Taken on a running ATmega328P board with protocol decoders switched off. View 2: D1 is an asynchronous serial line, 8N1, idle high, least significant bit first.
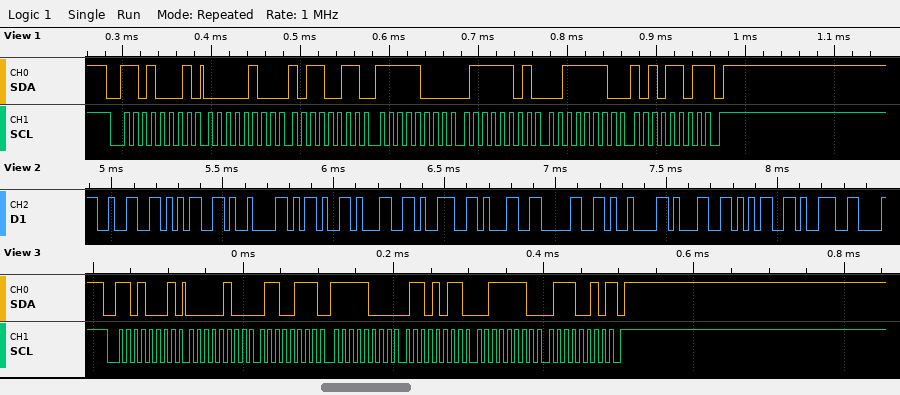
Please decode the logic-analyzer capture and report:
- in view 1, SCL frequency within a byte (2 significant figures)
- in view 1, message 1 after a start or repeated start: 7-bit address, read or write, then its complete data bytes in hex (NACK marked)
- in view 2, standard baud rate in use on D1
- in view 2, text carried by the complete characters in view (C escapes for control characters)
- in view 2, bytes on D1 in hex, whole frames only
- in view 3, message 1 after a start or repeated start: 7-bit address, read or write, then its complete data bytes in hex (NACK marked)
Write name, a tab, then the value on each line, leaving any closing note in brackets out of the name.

in view 1, SCL frequency within a byte	100 kHz
in view 1, message 1 after a start or repeated start: 7-bit address, read or write, then its complete data bytes in hex	0x68 read: 04 B3 F8 7D 3E AD NACK
in view 2, standard baud rate in use on D1	38400 baud
in view 2, text carried by the complete characters in view	"25\t-1910\t159"
in view 2, bytes on D1 in hex, whole frames only	32 35 09 2D 31 39 31 30 09 31 35 39
in view 3, message 1 after a start or repeated start: 7-bit address, read or write, then its complete data bytes in hex	0x68 read: 04 67 F8 6B 3E 72 NACK
